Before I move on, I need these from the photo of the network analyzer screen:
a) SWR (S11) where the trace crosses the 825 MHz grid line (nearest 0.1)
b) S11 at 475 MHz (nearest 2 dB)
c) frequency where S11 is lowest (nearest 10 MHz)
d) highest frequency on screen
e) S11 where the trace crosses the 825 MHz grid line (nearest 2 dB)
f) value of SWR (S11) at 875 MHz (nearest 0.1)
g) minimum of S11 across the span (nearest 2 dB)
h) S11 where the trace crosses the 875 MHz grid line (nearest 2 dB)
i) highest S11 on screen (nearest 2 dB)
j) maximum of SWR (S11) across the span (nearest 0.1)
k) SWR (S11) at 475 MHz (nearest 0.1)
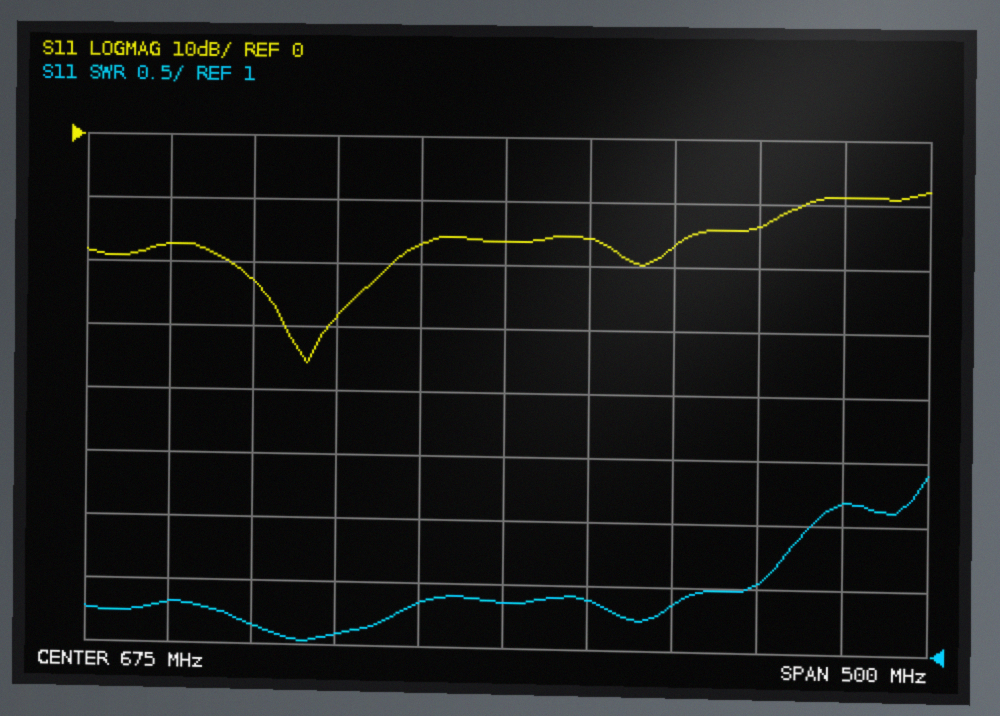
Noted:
1.5
-18 dB
560 MHz
925 MHz
-14 dB
2.2
-36 dB
-8 dB
-8 dB
2.4
1.3
